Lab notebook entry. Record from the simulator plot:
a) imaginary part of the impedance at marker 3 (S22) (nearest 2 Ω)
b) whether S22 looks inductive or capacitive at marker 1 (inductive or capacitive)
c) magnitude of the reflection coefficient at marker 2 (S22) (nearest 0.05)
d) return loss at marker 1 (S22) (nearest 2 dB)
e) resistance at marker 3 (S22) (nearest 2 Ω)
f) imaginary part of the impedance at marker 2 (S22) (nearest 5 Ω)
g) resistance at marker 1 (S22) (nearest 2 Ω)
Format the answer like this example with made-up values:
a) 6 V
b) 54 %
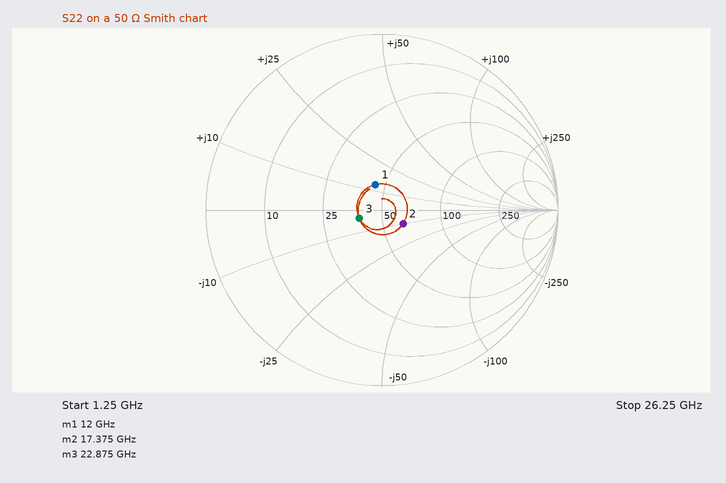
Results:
a) -4 Ω
b) inductive
c) 0.15
d) 16 dB
e) 38 Ω
f) -10 Ω
g) 44 Ω
